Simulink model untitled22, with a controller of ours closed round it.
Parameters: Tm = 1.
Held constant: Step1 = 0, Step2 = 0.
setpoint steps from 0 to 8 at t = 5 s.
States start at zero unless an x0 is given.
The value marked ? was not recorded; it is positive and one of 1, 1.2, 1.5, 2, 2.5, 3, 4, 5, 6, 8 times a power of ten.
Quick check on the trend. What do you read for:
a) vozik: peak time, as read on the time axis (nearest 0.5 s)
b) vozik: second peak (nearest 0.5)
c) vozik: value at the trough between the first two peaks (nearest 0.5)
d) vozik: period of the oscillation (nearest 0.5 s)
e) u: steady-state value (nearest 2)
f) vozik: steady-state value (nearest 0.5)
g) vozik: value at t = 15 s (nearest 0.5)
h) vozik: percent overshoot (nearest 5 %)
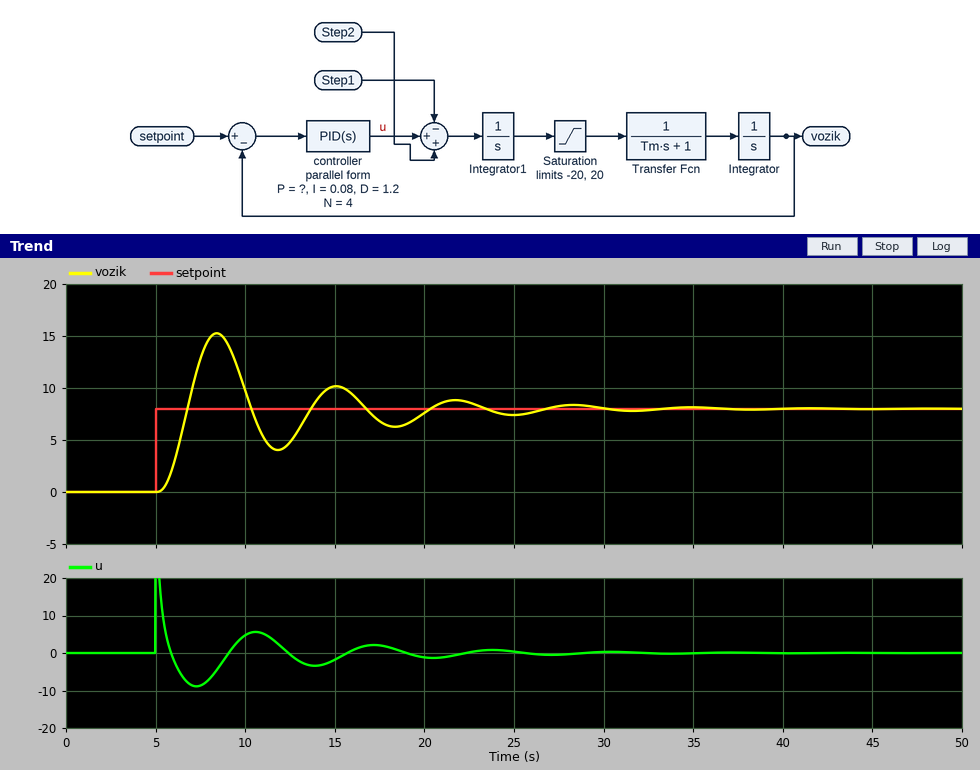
8.5 s
10.0
4.0
6.5 s
0
8.0
10.0
90 %
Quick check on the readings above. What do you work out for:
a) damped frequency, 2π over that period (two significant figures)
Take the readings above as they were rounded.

0.97 rad/s
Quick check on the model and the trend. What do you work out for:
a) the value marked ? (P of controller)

0.4
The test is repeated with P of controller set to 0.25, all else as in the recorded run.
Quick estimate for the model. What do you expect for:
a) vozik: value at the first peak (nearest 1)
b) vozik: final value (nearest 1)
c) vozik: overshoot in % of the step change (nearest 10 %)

14
8
80 %
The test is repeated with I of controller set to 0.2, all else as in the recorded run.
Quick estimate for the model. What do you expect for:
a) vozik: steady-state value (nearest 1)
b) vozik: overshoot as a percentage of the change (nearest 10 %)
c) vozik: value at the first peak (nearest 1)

8
110 %
17
